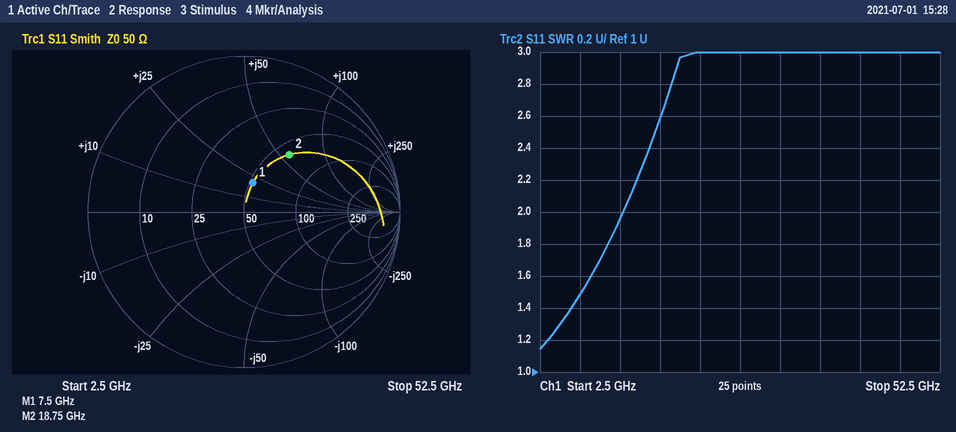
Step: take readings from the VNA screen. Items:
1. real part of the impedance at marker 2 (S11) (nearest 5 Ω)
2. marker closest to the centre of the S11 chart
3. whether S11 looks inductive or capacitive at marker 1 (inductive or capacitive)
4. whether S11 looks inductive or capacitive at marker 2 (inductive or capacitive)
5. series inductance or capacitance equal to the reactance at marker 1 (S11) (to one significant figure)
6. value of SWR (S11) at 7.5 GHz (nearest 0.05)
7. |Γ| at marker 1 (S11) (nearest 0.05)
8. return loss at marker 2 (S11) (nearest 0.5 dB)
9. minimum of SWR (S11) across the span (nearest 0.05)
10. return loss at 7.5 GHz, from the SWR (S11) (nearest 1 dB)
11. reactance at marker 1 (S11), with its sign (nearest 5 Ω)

60 Ω
marker 1
inductive
inductive
400 pH
1.50
0.20
6.5 dB
1.15
14 dB
+20 Ω
